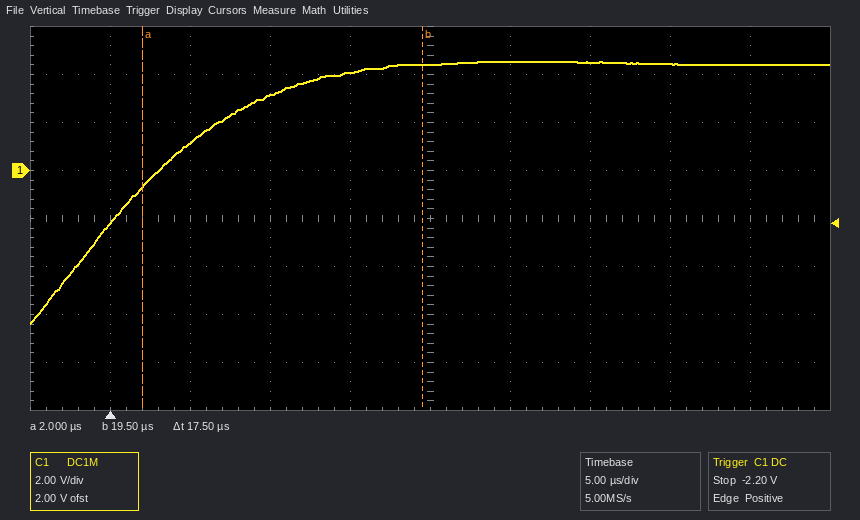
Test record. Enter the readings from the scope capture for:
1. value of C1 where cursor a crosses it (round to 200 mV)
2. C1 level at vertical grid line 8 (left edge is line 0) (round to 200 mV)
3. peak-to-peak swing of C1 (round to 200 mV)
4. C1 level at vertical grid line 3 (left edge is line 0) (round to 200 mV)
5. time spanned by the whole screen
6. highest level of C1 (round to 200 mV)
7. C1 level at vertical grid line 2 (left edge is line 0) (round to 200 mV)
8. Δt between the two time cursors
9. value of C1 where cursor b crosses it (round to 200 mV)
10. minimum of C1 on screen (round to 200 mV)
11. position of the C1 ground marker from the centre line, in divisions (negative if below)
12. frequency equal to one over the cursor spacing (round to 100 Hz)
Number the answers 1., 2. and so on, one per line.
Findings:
1. -600 mV
2. 4.4 V
3. 11.0 V
4. 3.2 V
5. 50 µs
6. 4.6 V
7. 1.2 V
8. 17.5 µs
9. 4.4 V
10. -6.4 V
11. +1.0 div
12. 57.1 kHz
